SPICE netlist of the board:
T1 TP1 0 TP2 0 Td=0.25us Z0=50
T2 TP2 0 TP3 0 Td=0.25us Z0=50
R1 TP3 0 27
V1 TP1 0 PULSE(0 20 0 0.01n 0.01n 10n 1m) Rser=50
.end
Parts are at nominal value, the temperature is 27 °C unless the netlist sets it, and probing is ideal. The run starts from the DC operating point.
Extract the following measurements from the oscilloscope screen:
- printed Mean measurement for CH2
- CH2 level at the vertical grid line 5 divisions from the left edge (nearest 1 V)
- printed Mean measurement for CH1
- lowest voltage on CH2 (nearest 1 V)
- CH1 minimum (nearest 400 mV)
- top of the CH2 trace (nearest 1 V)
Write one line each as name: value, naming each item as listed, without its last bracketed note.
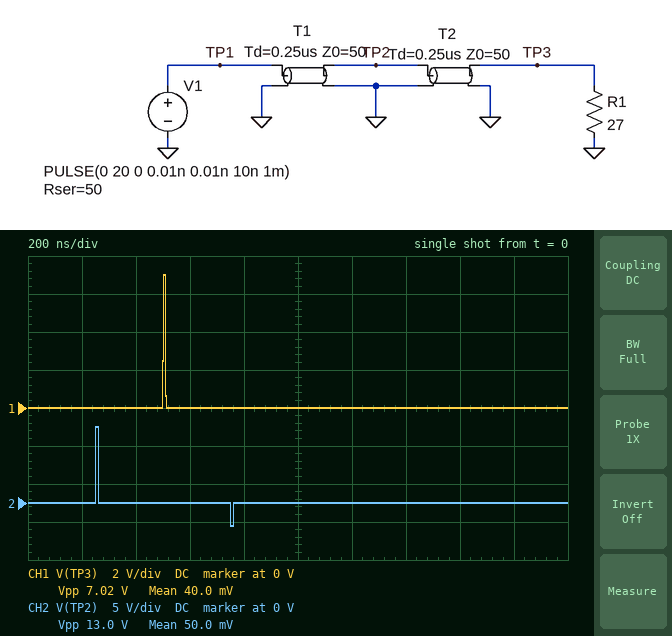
printed Mean measurement for CH2: 50.0 mV
CH2 level at the vertical grid line 5 divisions from the left edge: 0 V
printed Mean measurement for CH1: 40.0 mV
lowest voltage on CH2: -3 V
CH1 minimum: 0 V
top of the CH2 trace: 10 V
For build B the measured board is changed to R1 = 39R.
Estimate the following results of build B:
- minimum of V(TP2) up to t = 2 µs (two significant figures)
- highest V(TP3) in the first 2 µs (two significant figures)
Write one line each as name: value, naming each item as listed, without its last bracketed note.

minimum of V(TP2) up to t = 2 µs: -1.2 V
highest V(TP3) in the first 2 µs: 8.8 V
